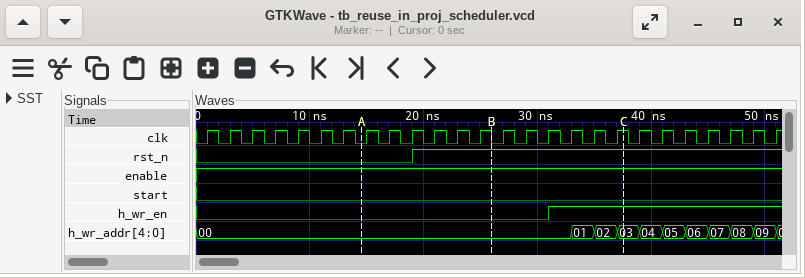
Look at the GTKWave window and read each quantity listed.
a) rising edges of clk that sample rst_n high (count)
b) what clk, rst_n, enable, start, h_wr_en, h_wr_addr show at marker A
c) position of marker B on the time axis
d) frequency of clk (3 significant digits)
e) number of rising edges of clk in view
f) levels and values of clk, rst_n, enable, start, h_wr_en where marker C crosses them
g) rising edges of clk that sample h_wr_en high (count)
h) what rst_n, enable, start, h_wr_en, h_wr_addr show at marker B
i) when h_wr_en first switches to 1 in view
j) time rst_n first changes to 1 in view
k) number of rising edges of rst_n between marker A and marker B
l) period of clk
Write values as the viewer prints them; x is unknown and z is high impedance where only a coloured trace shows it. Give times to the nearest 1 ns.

16
clk=0, rst_n=0, enable=1, start=0, h_wr_en=0, h_wr_addr=00
26 ns
500 MHz
26
clk=1, rst_n=1, enable=1, start=0, h_wr_en=1
10
rst_n=1, enable=1, start=0, h_wr_en=0, h_wr_addr=00
31 ns
19 ns
1
2 ns
